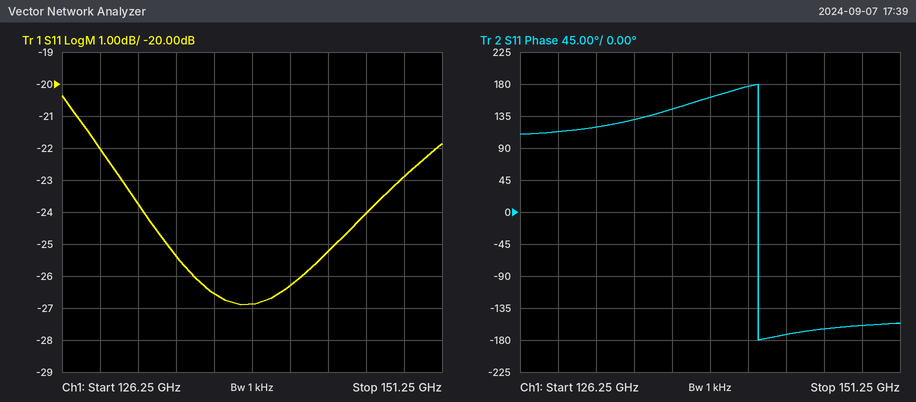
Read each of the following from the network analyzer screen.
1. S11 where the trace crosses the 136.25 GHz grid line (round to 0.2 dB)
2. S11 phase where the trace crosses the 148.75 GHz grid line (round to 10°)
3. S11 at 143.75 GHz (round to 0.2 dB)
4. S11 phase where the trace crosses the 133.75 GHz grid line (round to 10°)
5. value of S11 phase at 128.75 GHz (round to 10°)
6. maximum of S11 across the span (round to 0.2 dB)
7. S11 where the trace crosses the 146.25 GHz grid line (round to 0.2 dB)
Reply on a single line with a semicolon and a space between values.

-26.6 dB; -160°; -25.2 dB; 130°; 110°; -20.4 dB; -24.0 dB
